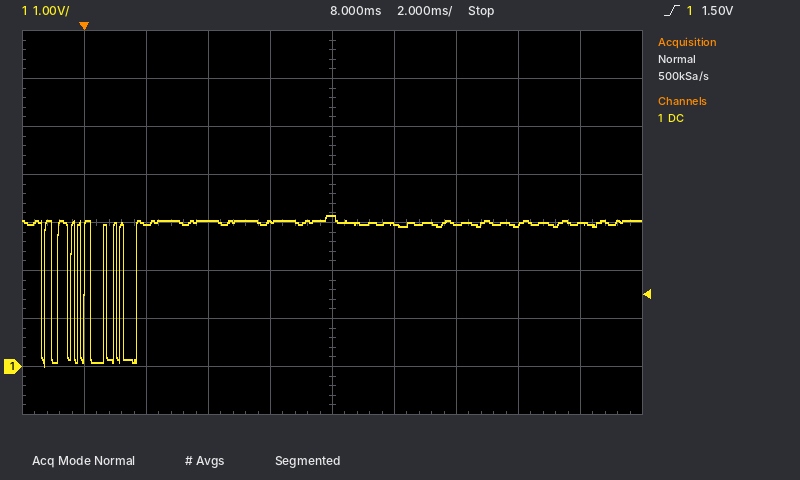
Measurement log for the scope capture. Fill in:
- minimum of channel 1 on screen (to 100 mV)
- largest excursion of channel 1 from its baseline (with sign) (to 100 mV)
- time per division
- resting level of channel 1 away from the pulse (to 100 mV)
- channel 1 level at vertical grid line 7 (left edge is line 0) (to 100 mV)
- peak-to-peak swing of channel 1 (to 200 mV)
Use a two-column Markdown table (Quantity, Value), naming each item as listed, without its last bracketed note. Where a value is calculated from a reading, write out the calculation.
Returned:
| Quantity | Value |
|---|---|
| minimum of channel 1 on screen | 0.0 V |
| largest excursion of channel 1 from its baseline (with sign) | 0.0 V − (3.0 V) = -3.0 V |
| time per division | 2 ms |
| resting level of channel 1 away from the pulse | 3.0 V |
| channel 1 level at vertical grid line 7 (left edge is line 0) | 3.0 V |
| peak-to-peak swing of channel 1 | 3.2 V |
